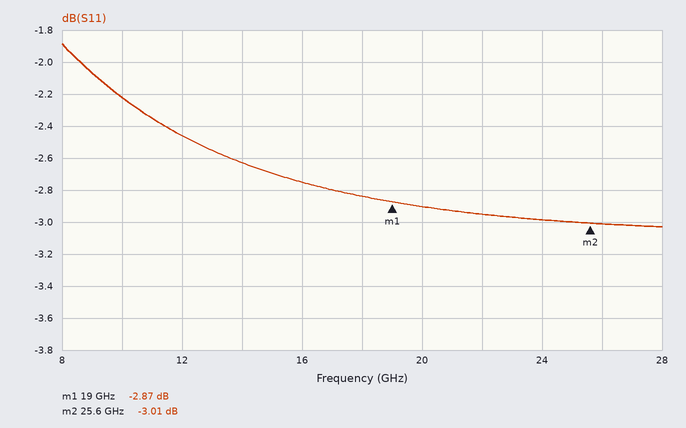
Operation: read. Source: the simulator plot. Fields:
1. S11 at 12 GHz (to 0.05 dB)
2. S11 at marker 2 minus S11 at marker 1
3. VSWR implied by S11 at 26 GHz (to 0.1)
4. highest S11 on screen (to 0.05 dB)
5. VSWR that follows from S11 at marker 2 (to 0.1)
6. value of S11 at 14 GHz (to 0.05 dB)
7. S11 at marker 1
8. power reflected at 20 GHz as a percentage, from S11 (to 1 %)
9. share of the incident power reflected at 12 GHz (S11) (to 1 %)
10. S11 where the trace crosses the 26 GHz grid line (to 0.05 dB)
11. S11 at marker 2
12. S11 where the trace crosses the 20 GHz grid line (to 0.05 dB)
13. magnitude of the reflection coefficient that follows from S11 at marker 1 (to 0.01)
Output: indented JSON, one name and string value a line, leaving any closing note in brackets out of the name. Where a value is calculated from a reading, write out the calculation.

{
  "S11 at 12 GHz": "-2.45 dB",
  "S11 at marker 2 minus S11 at marker 1": "-3.01 − (-2.87) = -0.14 dB",
  "VSWR implied by S11 at 26 GHz": "|Γ| = 10^(-3/20) = 0.7079; VSWR = (1 + 0.7079)/(1 − 0.7079) ≈ 5.8",
  "highest S11 on screen": "-1.90 dB",
  "VSWR that follows from S11 at marker 2": "(1 + 0.7071)/(1 − 0.7071) ≈ 5.8",
  "value of S11 at 14 GHz": "-2.65 dB",
  "S11 at marker 1": "-2.87 dB",
  "power reflected at 20 GHz as a percentage, from S11": "10^(-2.9/10) ≈ 51 %",
  "share of the incident power reflected at 12 GHz (S11)": "10^(-2.45/10) ≈ 57 %",
  "S11 where the trace crosses the 26 GHz grid line": "-3.00 dB",
  "S11 at marker 2": "-3.01 dB",
  "S11 where the trace crosses the 20 GHz grid line": "-2.90 dB",
  "magnitude of the reflection coefficient that follows from S11 at marker 1": "10^(-2.87/20) ≈ 0.72"
}
